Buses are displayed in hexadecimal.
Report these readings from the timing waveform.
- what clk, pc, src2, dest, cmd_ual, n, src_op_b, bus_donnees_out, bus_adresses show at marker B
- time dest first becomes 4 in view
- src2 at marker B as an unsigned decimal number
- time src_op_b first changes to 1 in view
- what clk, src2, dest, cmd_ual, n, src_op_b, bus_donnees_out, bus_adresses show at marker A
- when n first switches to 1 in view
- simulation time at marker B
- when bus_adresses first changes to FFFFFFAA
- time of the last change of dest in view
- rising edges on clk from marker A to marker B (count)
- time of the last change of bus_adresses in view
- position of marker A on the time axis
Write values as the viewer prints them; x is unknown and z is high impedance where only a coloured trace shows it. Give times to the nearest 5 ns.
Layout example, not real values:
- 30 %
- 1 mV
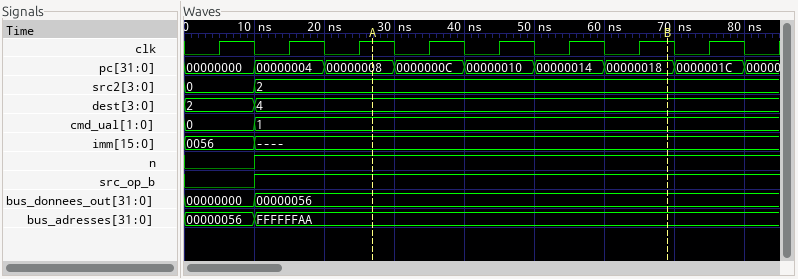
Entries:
- clk=1, pc=00000018, src2=2, dest=4, cmd_ual=1, n=1, src_op_b=1, bus_donnees_out=00000056, bus_adresses=FFFFFFAA
- 10 ns
- 2
- 10 ns
- clk=1, src2=2, dest=4, cmd_ual=1, n=1, src_op_b=1, bus_donnees_out=00000056, bus_adresses=FFFFFFAA
- 10 ns
- 70 ns
- 10 ns
- 10 ns
- 4
- 10 ns
- 25 ns
